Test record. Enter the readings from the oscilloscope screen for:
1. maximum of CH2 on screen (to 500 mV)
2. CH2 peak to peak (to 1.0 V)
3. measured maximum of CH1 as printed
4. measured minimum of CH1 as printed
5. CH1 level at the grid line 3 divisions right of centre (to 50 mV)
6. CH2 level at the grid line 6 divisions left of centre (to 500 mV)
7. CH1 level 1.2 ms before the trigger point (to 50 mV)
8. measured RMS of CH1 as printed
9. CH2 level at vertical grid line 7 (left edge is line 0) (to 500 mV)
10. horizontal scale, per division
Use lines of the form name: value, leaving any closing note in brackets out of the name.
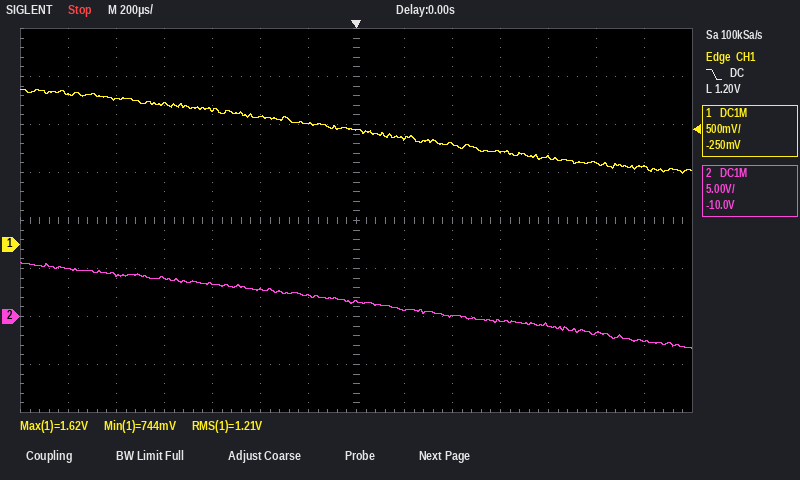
maximum of CH2 on screen: 5.5 V
CH2 peak to peak: 9.0 V
measured maximum of CH1 as printed: 1.62 V
measured minimum of CH1 as printed: 744 mV
CH1 level at the grid line 3 divisions right of centre: 950 mV
CH2 level at the grid line 6 divisions left of centre: 5.0 V
CH1 level 1.2 ms before the trigger point: 1.55 V
measured RMS of CH1 as printed: 1.21 V
CH2 level at vertical grid line 7 (left edge is line 0): 1.5 V
horizontal scale, per division: 200 µs
